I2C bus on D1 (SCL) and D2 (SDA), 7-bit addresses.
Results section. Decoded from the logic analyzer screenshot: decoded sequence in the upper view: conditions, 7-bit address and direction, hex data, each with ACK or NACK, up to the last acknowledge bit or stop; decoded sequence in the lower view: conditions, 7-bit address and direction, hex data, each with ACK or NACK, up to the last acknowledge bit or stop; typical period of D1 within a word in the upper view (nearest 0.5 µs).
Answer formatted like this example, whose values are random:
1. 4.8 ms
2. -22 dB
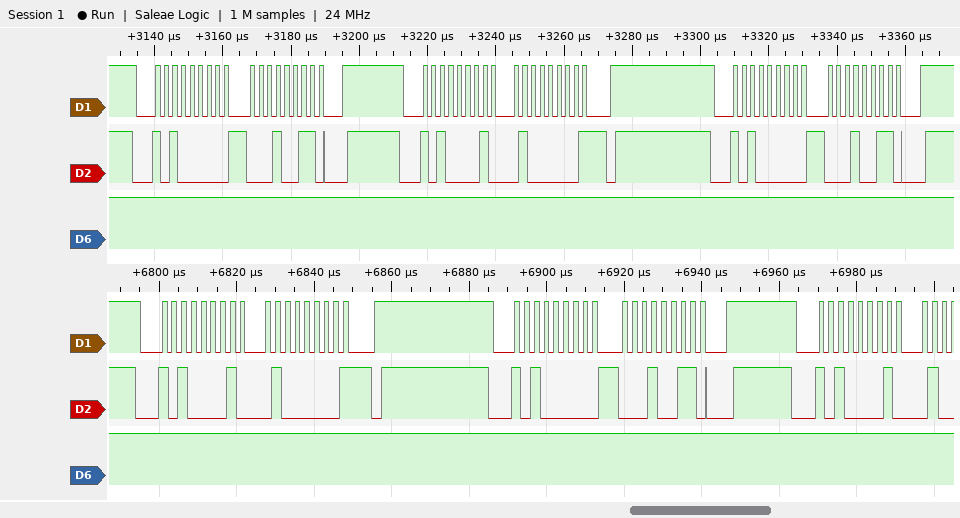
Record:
1. start, address 50 write ACK, 13 ACK, stop, start, address 50 read ACK, 40 NACK, stop, start, address 50 write ACK, 13 ACK, stop
2. start, address 50 read ACK, 40 NACK, stop, start, address 50 write ACK, 13 ACK, stop, start, address 50 read ACK
3. 2.5 µs
